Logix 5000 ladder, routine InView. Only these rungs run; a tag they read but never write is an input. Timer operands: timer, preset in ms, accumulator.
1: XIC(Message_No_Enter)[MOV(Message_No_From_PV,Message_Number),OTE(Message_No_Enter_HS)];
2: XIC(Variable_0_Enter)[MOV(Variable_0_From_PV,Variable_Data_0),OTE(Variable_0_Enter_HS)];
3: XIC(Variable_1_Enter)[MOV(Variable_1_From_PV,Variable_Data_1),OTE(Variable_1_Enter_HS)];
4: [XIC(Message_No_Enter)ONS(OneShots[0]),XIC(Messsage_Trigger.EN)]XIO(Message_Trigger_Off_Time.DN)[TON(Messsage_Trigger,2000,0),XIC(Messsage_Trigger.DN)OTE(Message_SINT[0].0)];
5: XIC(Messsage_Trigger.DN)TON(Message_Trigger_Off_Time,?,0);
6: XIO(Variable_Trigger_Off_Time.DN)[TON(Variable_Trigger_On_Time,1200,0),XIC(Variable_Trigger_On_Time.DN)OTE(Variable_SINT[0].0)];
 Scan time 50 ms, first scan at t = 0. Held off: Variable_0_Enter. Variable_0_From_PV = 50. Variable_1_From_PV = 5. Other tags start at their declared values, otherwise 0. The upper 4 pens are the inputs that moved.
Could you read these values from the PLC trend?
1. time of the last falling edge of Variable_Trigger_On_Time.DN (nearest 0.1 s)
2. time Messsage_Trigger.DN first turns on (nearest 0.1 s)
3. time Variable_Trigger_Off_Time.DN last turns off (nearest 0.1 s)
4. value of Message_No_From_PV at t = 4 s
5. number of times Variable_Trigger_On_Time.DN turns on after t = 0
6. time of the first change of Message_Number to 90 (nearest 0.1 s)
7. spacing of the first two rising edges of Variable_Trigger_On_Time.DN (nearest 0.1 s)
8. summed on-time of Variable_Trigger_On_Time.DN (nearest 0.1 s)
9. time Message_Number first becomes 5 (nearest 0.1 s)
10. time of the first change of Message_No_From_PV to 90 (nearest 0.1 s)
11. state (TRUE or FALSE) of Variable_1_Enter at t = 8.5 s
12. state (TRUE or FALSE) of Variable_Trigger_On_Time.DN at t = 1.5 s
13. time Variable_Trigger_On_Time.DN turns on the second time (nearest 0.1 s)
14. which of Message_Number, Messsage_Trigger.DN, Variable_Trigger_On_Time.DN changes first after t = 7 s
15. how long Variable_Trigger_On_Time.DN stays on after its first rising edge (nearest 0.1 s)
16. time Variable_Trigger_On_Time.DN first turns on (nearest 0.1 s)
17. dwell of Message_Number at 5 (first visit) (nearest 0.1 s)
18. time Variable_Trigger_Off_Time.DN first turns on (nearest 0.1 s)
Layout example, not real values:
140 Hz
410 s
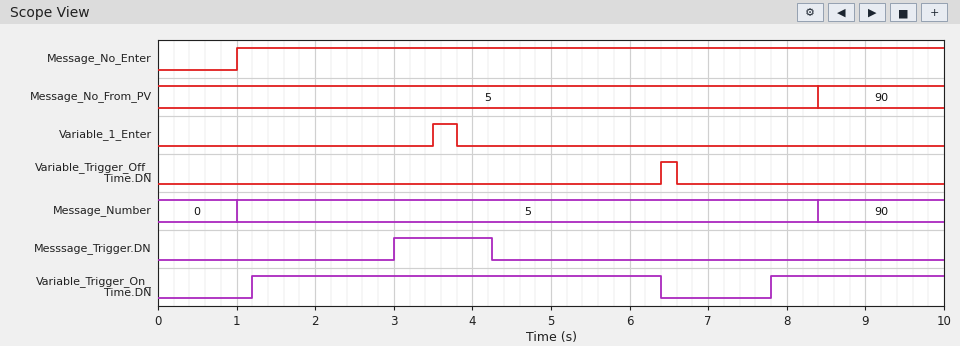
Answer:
6.4 s
3.0 s
6.6 s
5
2
8.4 s
6.6 s
7.4 s
1.0 s
8.4 s
FALSE
TRUE
7.8 s
Variable_Trigger_On_Time.DN
5.2 s
1.2 s
7.4 s
6.4 s
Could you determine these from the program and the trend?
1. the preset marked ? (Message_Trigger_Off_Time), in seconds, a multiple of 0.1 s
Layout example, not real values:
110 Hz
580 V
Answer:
1.2 s
